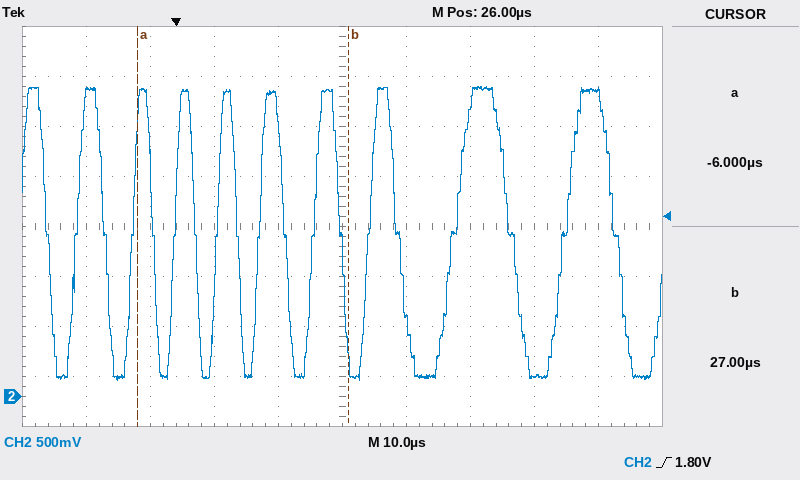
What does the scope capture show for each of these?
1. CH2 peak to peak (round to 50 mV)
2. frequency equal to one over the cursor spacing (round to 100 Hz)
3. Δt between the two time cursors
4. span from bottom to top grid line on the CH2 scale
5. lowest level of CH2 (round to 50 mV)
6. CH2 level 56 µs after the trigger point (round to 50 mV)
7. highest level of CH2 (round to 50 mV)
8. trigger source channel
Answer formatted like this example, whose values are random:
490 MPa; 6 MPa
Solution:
2.95 V; 30.3 kHz; 33 µs; 4 V; 150 mV; 200 mV; 3.10 V; CH2
